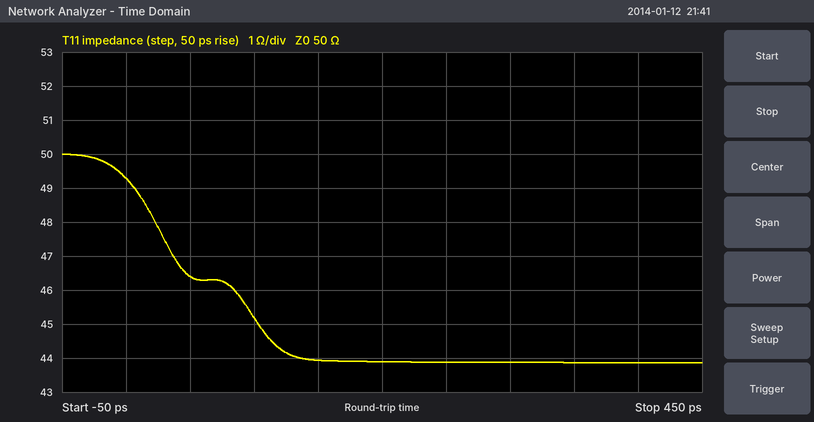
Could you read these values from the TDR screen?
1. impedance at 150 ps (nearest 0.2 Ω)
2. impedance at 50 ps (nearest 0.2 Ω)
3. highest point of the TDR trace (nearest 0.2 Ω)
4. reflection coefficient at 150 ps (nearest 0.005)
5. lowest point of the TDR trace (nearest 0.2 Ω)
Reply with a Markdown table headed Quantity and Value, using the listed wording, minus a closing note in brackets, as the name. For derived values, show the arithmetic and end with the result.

| Quantity | Value |
|---|---|
| impedance at 150 ps | 44.0 Ω |
| impedance at 50 ps | 46.4 Ω |
| highest point of the TDR trace | 50.0 Ω |
| reflection coefficient at 150 ps | (44 − 50)/(44 + 50) ≈ -0.0638, so -0.065 to the nearest 0.005 |
| lowest point of the TDR trace | 43.8 Ω |
